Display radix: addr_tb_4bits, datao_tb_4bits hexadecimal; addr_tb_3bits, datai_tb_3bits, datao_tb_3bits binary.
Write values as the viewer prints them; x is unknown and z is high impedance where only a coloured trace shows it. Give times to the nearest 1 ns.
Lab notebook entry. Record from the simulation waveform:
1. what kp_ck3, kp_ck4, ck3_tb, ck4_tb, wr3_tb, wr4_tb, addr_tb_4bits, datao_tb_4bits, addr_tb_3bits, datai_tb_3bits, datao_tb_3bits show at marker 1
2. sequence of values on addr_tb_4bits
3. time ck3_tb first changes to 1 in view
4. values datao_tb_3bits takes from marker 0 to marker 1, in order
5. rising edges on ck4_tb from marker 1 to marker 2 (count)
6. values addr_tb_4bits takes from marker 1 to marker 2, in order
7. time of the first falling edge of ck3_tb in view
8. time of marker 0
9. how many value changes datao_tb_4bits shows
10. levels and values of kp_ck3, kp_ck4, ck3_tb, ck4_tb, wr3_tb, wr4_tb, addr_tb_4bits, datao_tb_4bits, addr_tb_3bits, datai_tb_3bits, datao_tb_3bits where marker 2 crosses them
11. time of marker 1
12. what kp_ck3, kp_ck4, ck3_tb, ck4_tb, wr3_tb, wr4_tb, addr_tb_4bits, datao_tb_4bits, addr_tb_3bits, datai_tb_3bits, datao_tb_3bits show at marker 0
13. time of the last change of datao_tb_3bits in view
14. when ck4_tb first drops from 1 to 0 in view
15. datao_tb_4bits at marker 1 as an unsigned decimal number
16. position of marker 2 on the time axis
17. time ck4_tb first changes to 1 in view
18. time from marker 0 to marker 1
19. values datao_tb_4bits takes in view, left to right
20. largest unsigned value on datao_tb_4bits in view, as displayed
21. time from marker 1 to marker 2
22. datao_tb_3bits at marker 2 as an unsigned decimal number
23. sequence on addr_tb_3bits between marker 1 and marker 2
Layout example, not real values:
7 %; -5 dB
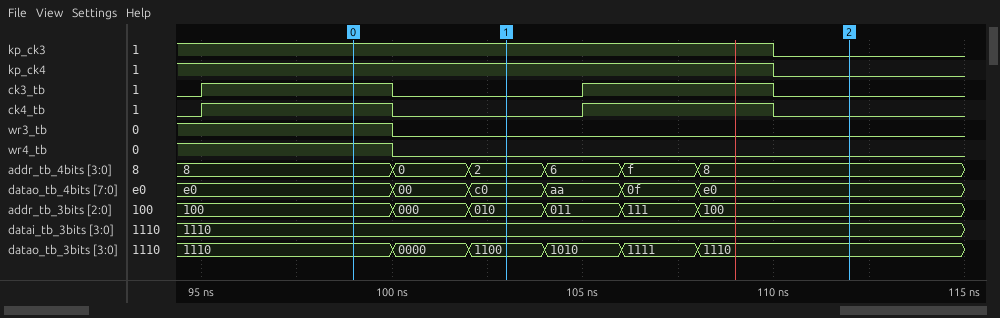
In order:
kp_ck3=1, kp_ck4=1, ck3_tb=0, ck4_tb=0, wr3_tb=0, wr4_tb=0, addr_tb_4bits=2, datao_tb_4bits=c0, addr_tb_3bits=010, datai_tb_3bits=1110, datao_tb_3bits=1100; 8, 0, 2, 6, f, 8; 95 ns; 1110, 0000, 1100; 1; 2, 6, f, 8; 100 ns; 99 ns; 5; kp_ck3=0, kp_ck4=0, ck3_tb=0, ck4_tb=0, wr3_tb=0, wr4_tb=0, addr_tb_4bits=8, datao_tb_4bits=e0, addr_tb_3bits=100, datai_tb_3bits=1110, datao_tb_3bits=1110; 103 ns; kp_ck3=1, kp_ck4=1, ck3_tb=1, ck4_tb=1, wr3_tb=1, wr4_tb=1, addr_tb_4bits=8, datao_tb_4bits=e0, addr_tb_3bits=100, datai_tb_3bits=1110, datao_tb_3bits=1110; 108 ns; 100 ns; 192; 112 ns; 95 ns; 4 ns; e0, 00, c0, aa, 0f, e0; e0; 9 ns; 14; 010, 011, 111, 100
